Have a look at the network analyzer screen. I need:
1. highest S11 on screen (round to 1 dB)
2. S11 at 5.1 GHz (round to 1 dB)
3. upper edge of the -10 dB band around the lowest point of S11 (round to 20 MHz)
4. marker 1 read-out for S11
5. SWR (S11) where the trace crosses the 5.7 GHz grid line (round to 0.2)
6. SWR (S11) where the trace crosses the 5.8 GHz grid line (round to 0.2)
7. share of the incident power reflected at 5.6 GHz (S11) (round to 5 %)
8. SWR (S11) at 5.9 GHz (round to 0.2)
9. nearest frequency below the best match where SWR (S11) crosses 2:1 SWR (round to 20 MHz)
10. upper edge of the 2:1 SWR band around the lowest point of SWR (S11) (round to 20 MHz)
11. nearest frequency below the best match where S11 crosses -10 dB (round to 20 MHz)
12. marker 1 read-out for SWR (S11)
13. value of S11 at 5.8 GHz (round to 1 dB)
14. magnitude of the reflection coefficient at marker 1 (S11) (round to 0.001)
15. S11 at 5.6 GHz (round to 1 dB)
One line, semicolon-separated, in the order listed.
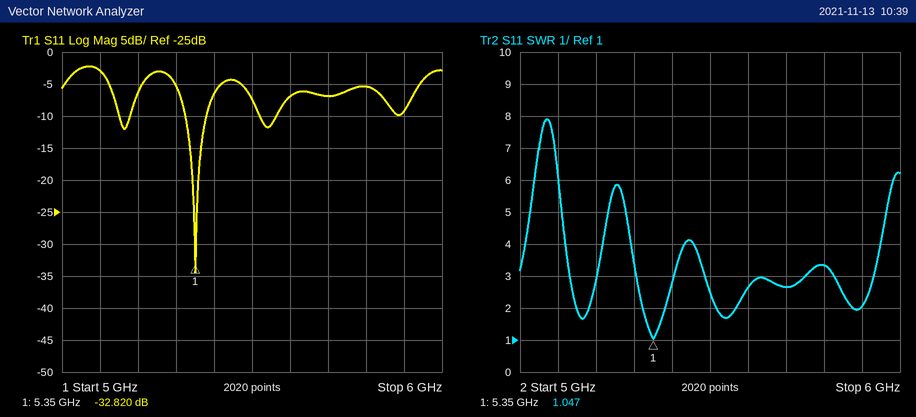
-2 dB; -3 dB; 5.38 GHz; -32.820 dB; 2.6; 3.4; 20 %; 2.0; 5.32 GHz; 5.38 GHz; 5.32 GHz; 1.047; -5 dB; 0.023; -7 dB
